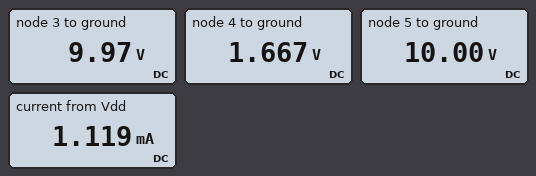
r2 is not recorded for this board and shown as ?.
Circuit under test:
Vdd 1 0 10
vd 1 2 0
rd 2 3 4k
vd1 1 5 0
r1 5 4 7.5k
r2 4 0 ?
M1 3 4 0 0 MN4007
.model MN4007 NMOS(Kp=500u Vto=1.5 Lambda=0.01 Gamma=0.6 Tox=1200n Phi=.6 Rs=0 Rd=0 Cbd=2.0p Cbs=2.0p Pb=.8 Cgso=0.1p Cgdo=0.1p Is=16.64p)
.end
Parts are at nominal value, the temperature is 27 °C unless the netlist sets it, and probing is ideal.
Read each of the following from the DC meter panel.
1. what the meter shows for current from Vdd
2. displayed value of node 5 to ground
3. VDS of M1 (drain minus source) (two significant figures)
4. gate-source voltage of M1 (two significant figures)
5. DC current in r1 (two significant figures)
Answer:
1.119 mA
10.00 V
10 V
1.7 V
1.1 mA
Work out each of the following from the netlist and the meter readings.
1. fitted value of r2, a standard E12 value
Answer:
1.5 kΩ
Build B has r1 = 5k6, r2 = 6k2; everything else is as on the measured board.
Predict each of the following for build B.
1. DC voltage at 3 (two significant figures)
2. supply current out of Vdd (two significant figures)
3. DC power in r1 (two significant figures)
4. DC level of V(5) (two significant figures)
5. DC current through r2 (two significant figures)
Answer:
1.4 V
3.0 mA
4.0 mW
10 V
850 µA
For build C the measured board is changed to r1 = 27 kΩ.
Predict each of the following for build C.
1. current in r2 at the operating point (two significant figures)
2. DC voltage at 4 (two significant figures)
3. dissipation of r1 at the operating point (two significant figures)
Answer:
350 µA
530 mV
3.3 mW
